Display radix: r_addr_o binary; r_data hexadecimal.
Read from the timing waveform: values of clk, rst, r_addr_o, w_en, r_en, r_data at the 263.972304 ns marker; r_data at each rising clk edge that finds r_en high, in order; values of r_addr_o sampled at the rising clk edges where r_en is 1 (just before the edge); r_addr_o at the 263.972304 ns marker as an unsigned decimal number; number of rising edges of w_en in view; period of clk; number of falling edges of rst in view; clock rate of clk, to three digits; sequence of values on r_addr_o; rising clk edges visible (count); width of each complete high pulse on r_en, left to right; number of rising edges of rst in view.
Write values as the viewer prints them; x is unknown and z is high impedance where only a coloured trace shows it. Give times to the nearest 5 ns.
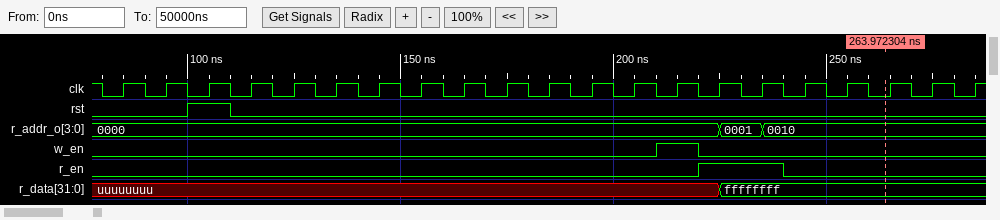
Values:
clk=0, rst=0, r_addr_o=0010, w_en=0, r_en=0, r_data=ffffffff
uuuuuuuu, ffffffff
0000, 0001
2
1
10 ns
1
100 MHz
0000, 0001, 0010
21
20 ns
1
